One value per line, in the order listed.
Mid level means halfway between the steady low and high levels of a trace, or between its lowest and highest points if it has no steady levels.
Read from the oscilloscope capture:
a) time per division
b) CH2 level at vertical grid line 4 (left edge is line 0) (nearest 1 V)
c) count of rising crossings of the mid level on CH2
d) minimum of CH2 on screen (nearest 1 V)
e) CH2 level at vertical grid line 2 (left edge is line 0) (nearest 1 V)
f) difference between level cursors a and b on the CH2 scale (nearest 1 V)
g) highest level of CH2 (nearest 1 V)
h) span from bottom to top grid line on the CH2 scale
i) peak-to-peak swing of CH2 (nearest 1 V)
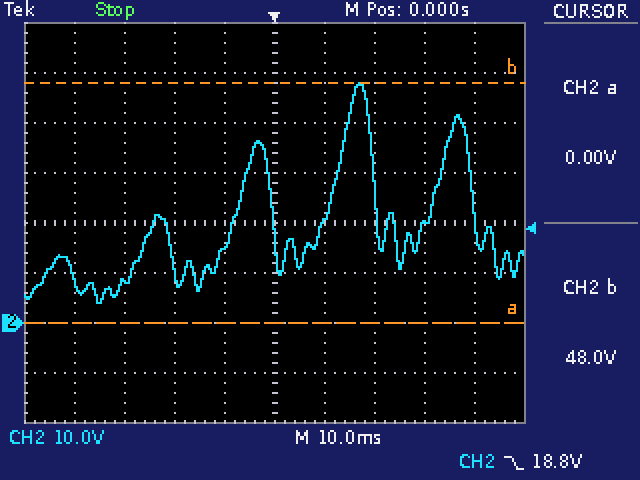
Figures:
10 ms
15 V
3
4 V
8 V
48 V
48 V
80 V
44 V
